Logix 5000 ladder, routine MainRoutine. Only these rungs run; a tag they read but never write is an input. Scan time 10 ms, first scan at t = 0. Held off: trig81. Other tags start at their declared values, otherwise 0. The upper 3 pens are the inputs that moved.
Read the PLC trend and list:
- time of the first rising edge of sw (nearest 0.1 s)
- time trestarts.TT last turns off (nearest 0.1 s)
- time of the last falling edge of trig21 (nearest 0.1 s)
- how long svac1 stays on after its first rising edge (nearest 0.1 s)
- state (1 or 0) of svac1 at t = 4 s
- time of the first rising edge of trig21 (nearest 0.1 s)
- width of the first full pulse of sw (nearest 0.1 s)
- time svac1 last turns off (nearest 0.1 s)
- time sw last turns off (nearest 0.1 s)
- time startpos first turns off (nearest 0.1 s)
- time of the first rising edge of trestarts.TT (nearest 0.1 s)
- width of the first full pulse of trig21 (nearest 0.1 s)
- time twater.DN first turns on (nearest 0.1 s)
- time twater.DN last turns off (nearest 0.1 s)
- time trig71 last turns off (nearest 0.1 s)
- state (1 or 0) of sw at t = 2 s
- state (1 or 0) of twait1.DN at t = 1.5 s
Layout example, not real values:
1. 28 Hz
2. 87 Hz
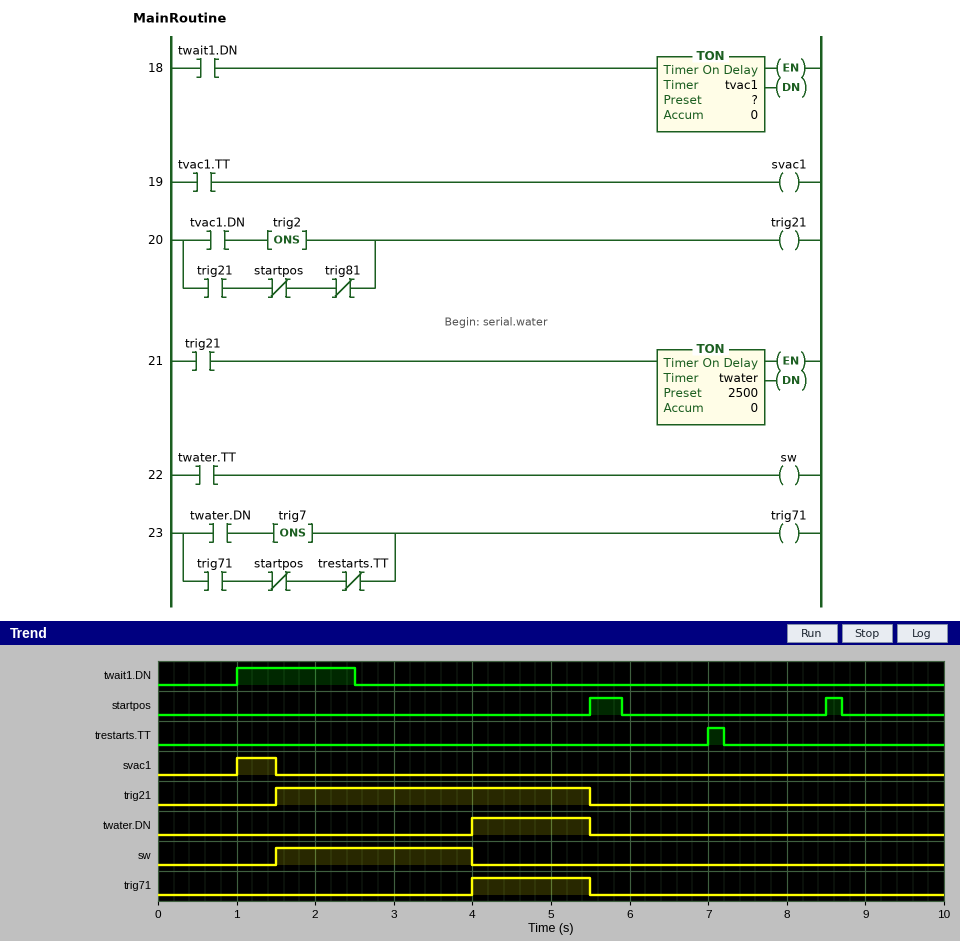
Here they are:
1. 1.5 s
2. 7.2 s
3. 5.5 s
4. 0.5 s
5. 0
6. 1.5 s
7. 2.5 s
8. 1.5 s
9. 4.0 s
10. 5.9 s
11. 7.0 s
12. 4.0 s
13. 4.0 s
14. 5.5 s
15. 5.5 s
16. 1
17. 1
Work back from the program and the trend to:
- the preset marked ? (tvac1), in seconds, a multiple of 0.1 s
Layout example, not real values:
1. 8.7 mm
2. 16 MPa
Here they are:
1. 0.5 s
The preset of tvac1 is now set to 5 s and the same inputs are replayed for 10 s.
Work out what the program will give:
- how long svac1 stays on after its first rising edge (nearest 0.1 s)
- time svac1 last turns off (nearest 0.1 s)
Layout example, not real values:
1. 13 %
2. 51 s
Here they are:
1. 1.5 s
2. 2.5 s
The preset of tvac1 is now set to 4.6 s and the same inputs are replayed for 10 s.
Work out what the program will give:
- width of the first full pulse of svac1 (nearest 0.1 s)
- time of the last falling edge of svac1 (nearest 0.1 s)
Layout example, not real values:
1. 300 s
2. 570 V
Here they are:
1. 1.5 s
2. 2.5 s
